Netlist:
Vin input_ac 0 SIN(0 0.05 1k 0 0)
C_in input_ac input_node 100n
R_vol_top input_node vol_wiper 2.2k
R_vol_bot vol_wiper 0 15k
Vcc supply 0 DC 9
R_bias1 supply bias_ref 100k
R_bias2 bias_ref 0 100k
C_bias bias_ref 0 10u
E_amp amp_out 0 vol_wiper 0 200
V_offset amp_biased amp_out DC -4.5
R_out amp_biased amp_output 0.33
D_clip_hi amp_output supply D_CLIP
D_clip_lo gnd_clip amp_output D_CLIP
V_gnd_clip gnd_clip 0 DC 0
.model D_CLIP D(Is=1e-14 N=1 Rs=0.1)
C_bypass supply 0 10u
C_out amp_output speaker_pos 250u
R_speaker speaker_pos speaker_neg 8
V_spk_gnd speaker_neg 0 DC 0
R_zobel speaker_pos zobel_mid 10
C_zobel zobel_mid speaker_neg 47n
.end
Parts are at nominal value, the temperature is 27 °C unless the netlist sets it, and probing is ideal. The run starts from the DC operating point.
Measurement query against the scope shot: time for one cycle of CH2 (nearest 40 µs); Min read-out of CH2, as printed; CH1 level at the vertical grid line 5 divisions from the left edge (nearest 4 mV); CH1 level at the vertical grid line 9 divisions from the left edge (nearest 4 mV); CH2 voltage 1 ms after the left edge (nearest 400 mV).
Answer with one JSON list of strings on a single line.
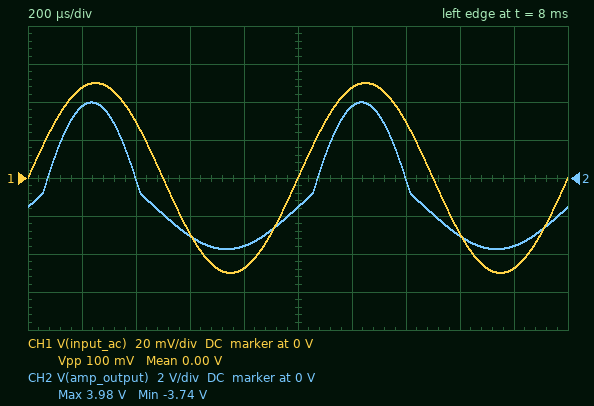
["1.00 ms", "-3.74 V", "0 V", "-48 mV", "-1.6 V"]
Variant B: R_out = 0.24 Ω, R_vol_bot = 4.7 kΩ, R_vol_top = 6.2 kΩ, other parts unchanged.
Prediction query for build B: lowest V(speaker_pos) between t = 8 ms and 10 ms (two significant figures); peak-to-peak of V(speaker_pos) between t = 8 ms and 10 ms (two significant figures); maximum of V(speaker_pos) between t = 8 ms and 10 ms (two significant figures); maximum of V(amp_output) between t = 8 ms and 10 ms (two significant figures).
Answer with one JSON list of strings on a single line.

["-1.3 V", "2.9 V", "1.6 V", "-280 mV"]
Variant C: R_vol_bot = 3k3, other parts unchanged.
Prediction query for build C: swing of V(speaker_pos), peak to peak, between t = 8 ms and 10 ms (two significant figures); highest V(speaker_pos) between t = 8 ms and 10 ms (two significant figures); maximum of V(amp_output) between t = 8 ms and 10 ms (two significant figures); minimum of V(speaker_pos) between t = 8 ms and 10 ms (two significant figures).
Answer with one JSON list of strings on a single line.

["4.2 V", "2.6 V", "1.2 V", "-1.6 V"]
